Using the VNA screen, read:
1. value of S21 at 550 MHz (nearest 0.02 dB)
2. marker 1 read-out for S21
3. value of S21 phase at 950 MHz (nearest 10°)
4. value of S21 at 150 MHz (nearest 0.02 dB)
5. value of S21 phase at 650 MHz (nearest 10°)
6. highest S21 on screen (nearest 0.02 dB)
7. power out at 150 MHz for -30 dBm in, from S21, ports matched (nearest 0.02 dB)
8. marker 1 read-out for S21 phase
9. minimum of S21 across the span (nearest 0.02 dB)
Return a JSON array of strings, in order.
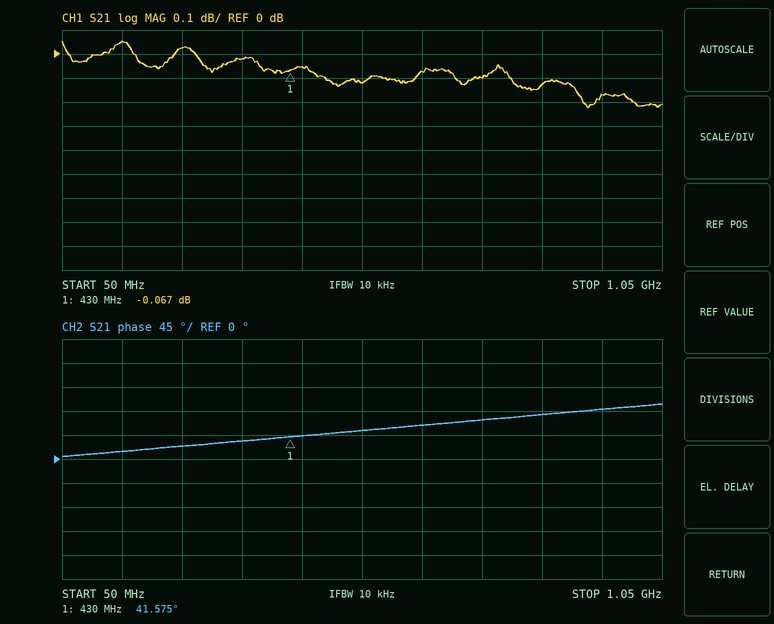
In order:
["-0.12 dB", "-0.067 dB", "90°", "0.06 dB", "60°", "0.06 dB", "-29.94 dBm", "41.575°", "-0.22 dB"]
